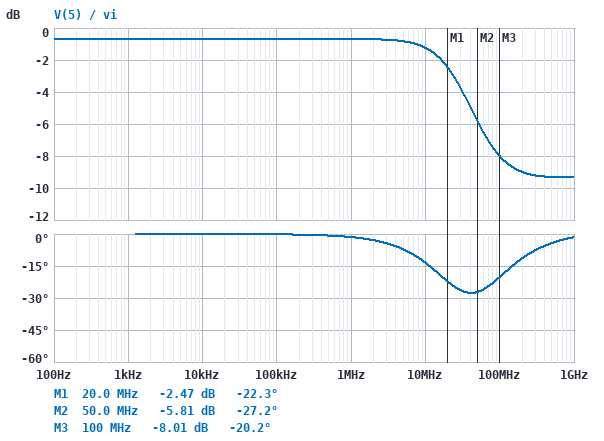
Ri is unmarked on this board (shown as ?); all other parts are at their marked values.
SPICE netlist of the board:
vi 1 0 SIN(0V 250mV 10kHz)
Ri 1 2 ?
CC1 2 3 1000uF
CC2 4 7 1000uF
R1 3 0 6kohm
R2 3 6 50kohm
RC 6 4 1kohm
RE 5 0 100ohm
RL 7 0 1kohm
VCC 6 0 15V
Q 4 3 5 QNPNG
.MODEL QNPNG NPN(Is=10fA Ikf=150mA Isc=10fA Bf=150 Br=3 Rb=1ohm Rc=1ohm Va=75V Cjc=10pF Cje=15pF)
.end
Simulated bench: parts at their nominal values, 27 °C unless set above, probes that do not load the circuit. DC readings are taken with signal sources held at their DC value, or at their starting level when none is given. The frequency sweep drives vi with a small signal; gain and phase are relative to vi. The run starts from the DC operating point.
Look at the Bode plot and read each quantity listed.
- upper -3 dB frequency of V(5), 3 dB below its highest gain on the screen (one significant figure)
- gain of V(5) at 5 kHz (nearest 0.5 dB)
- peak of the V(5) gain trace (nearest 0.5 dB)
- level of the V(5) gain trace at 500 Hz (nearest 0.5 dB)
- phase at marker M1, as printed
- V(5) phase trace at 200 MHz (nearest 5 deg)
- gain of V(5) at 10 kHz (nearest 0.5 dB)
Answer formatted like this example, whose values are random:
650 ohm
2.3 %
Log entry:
30 MHz
-0.5 dB
-0.5 dB
-0.5 dB
-22.3 deg
-10 deg
-0.5 dB
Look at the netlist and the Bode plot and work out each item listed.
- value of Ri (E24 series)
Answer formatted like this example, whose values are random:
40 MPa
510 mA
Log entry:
150 Ω
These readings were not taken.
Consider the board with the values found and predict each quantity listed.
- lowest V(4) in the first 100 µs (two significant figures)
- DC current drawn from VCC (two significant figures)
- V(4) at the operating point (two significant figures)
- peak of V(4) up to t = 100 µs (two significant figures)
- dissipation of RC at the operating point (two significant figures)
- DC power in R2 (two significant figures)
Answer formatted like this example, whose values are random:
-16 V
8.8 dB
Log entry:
7.1 V
7.0 mA
8.3 V
9.4 V
45 mW
3.7 mW
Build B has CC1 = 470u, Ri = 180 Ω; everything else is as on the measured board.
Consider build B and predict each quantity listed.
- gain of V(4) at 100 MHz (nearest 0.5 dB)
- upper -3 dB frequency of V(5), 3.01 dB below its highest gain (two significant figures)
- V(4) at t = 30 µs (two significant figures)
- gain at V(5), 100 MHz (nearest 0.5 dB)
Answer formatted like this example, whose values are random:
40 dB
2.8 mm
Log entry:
0.5 dB
25 MHz
7.2 V
-9.0 dB
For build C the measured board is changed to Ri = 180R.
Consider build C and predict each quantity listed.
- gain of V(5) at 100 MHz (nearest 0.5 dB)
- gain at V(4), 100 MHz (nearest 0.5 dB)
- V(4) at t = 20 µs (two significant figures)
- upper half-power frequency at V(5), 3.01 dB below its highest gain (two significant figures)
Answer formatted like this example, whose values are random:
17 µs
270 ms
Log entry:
-9.0 dB
0.5 dB
7.2 V
25 MHz
